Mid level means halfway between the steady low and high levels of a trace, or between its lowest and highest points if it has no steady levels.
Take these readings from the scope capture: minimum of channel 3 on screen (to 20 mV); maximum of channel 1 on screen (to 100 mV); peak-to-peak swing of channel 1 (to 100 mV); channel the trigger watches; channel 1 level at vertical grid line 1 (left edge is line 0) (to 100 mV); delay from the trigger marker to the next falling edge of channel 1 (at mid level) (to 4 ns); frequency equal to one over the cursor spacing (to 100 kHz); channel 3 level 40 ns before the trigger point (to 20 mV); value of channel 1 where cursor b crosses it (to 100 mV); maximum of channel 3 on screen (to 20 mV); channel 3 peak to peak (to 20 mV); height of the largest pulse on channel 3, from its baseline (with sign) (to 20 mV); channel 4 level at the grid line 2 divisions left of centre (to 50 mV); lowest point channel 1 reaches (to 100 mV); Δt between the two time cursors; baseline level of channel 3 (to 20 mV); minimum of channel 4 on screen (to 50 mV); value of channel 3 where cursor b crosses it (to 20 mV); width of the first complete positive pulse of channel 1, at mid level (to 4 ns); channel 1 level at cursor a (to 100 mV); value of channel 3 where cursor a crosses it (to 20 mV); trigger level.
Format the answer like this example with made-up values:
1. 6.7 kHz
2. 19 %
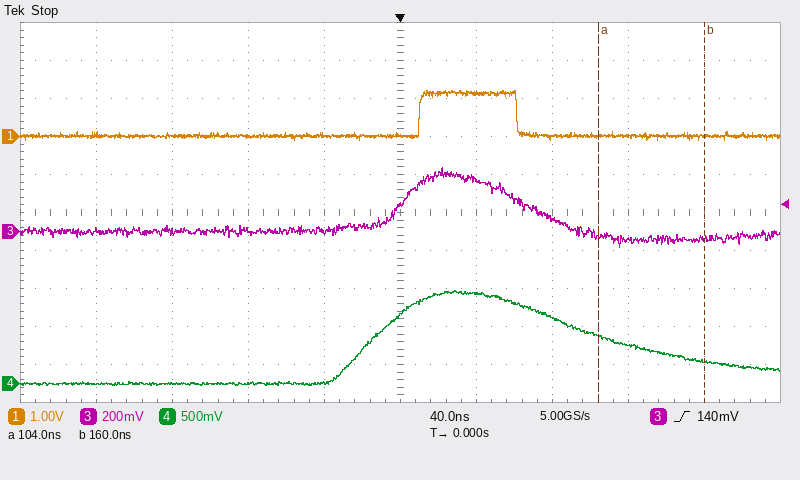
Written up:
1. -80 mV
2. 1.2 V
3. 1.3 V
4. channel 3
5. 0.0 V
6. 60 ns
7. 17.9 MHz
8. 0 mV
9. 0.0 V
10. 340 mV
11. 420 mV
12. +340 mV
13. 0 mV
14. -100 mV
15. 56 ns
16. 0 mV
17. -50 mV
18. -40 mV
19. 52 ns
20. 0.0 V
21. -20 mV
22. 140 mV
